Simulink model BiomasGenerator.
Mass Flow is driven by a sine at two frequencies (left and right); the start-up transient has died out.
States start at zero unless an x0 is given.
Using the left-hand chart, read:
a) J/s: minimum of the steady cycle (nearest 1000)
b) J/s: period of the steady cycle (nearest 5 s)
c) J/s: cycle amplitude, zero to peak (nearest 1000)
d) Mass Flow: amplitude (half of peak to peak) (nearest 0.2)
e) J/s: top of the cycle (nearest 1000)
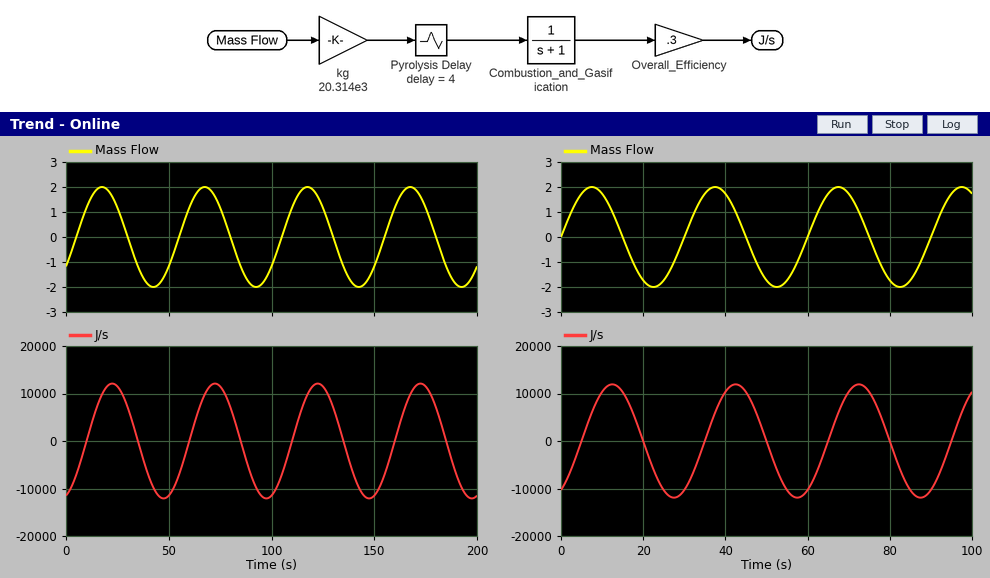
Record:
-12000
50 s
12000
2.0
12000
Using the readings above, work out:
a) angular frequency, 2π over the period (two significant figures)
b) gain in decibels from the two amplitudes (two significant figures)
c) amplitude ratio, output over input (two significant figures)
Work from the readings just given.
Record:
0.13 rad/s
76 dB
6000
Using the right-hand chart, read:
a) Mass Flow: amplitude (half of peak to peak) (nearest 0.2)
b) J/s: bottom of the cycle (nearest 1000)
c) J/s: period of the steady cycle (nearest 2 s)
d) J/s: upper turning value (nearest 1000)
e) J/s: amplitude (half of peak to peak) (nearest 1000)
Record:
2.0
-12000
30 s
12000
12000
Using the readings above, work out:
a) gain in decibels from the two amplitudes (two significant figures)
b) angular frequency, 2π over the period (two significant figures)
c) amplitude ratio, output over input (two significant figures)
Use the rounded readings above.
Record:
76 dB
0.21 rad/s
6000
